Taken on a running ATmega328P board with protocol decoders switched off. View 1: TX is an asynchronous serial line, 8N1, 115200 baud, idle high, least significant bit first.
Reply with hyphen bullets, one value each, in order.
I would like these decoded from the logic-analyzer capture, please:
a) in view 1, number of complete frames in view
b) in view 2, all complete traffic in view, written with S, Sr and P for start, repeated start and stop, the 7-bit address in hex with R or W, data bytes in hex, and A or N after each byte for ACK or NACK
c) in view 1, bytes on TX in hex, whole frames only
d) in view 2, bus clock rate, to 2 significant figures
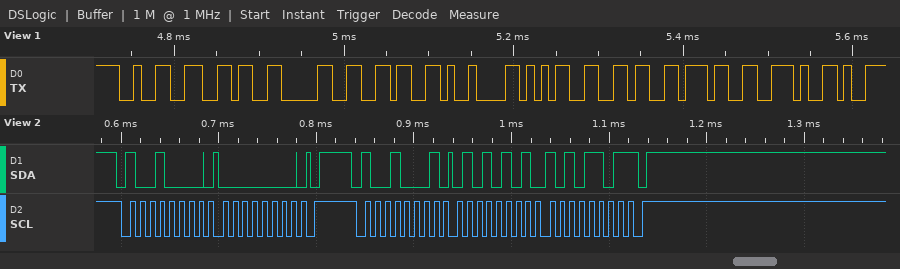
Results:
- 9
- S 48W A 00 A P S 48R A 55 A AD N P
- 32 36 30 36 09 35 36 37 2E
- 100 kHz
